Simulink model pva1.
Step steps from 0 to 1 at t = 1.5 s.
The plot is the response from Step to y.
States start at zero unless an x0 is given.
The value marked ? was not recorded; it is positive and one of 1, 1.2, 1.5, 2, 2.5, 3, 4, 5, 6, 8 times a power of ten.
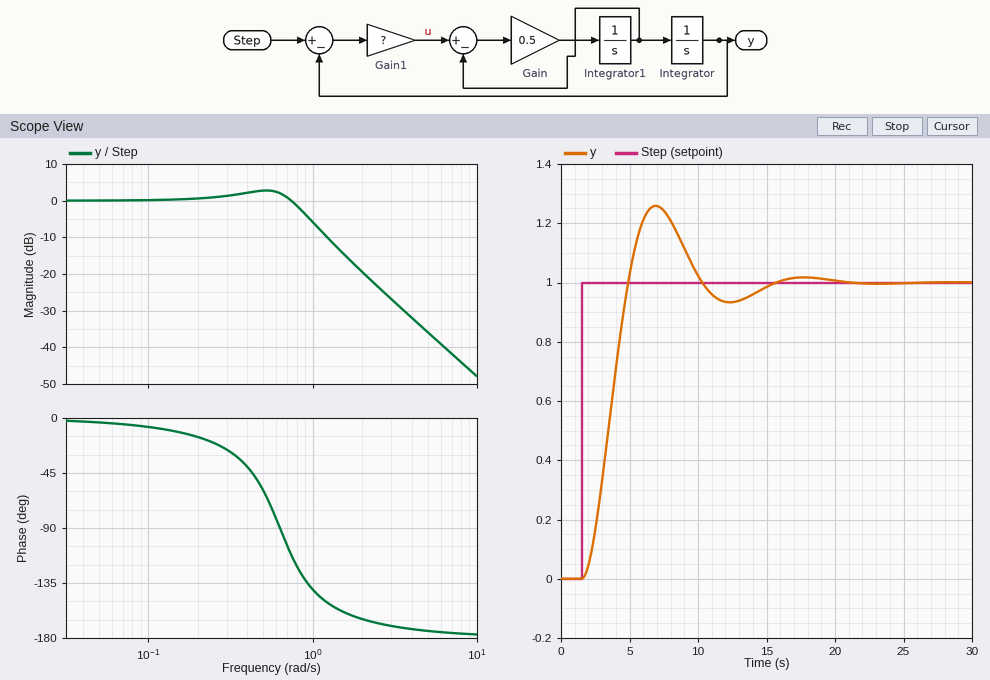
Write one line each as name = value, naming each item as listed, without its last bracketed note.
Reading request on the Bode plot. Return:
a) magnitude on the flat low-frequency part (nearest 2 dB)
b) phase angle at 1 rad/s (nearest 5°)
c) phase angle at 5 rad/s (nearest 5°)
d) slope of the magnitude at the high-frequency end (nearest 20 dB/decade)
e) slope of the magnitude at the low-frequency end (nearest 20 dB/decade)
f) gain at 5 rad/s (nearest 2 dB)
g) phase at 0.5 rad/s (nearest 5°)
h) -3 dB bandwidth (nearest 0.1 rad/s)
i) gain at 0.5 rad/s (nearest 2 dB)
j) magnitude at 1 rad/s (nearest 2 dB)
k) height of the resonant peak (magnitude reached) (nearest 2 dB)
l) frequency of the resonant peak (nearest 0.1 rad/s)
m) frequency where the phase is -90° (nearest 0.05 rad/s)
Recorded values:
magnitude on the flat low-frequency part = 0 dB
phase angle at 1 rad/s = -140°
phase angle at 5 rad/s = -175°
slope of the magnitude at the high-frequency end = -40 dB/decade
slope of the magnitude at the low-frequency end = 0 dB/decade
gain at 5 rad/s = -36 dB
phase at 0.5 rad/s = -60°
-3 dB bandwidth = 0.9 rad/s
gain at 0.5 rad/s = 2 dB
magnitude at 1 rad/s = -6 dB
height of the resonant peak (magnitude reached) = 2 dB
frequency of the resonant peak = 0.5 rad/s
frequency where the phase is -90° = 0.65 rad/s
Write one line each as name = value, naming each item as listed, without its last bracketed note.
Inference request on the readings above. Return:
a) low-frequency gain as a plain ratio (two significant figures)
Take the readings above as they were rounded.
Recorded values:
low-frequency gain as a plain ratio = 1.0
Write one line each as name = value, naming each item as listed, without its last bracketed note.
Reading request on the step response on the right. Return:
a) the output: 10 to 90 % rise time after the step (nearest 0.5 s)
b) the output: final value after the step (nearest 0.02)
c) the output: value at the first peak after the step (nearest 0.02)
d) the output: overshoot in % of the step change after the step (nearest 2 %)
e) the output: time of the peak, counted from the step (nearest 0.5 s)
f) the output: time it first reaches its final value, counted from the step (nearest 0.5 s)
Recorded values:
the output: 10 to 90 % rise time after the step = 2.5 s
the output: final value after the step = 1.00
the output: value at the first peak after the step = 1.26
the output: overshoot in % of the step change after the step = 26 %
the output: time of the peak, counted from the step = 5.5 s
the output: time it first reaches its final value, counted from the step = 3.5 s
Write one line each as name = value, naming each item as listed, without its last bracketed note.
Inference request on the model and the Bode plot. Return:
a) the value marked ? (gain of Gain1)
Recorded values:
the value marked ? = 0.8
